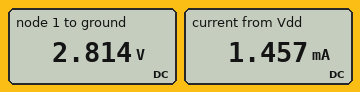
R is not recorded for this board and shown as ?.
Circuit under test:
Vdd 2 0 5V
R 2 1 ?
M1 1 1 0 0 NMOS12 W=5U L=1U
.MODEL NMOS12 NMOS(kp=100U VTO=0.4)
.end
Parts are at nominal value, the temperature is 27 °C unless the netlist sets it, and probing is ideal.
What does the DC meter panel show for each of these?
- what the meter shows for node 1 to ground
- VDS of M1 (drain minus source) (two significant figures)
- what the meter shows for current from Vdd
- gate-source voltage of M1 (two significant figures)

2.814 V
2.8 V
1.457 mA
2.8 V
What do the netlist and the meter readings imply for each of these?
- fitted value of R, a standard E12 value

1.5 kΩ
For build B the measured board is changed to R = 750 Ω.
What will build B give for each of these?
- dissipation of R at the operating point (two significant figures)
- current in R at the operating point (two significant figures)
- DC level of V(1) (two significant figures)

3.6 mW
2.2 mA
3.4 V
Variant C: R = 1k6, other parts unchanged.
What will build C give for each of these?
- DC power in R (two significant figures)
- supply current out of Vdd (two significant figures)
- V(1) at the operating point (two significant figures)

3.1 mW
1.4 mA
2.8 V
